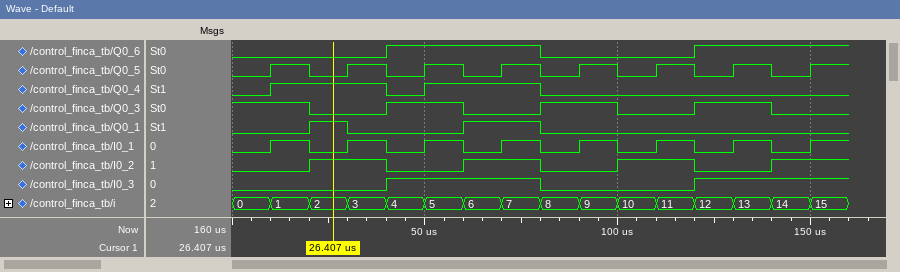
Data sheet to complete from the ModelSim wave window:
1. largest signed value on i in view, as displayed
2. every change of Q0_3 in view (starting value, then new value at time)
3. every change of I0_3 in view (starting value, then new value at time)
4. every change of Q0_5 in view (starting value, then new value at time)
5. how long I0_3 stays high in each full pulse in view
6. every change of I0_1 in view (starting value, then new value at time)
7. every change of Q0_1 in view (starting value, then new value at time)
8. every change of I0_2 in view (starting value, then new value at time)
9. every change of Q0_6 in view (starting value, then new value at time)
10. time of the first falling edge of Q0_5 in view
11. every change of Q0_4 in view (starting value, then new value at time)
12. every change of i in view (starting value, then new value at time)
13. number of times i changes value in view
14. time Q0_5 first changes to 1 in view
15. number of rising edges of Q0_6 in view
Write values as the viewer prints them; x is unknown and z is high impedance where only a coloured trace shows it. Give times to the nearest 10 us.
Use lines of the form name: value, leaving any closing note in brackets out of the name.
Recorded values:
largest signed value on i in view, as displayed: 15
every change of Q0_3 in view: 1, 0 at 20 us, 1 at 40 us, 0 at 60 us, 1 at 80 us, 0 at 100 us, 1 at 120 us, 0 at 140 us
every change of I0_3 in view: 0, 1 at 40 us, 0 at 80 us, 1 at 120 us
every change of Q0_5 in view: 0, 1 at 10 us, 0 at 20 us, 1 at 30 us, 0 at 40 us, 1 at 50 us, 0 at 60 us, 1 at 70 us, 0 at 80 us, 1 at 90 us, 0 at 100 us, 1 at 110 us, 0 at 120 us, 1 at 130 us, 0 at 140 us, 1 at 150 us
how long I0_3 stays high in each full pulse in view: 40 us
every change of I0_1 in view: 0, 1 at 10 us, 0 at 20 us, 1 at 30 us, 0 at 40 us, 1 at 50 us, 0 at 60 us, 1 at 70 us, 0 at 80 us, 1 at 90 us, 0 at 100 us, 1 at 110 us, 0 at 120 us, 1 at 130 us, 0 at 140 us, 1 at 150 us
every change of Q0_1 in view: 0, 1 at 20 us, 0 at 30 us, 1 at 60 us, 0 at 80 us
every change of I0_2 in view: 0, 1 at 20 us, 0 at 40 us, 1 at 60 us, 0 at 80 us, 1 at 100 us, 0 at 120 us, 1 at 140 us
every change of Q0_6 in view: 0, 1 at 40 us, 0 at 80 us, 1 at 120 us
time of the first falling edge of Q0_5 in view: 20 us
every change of Q0_4 in view: 0, 1 at 10 us, 0 at 40 us, 1 at 50 us, 0 at 80 us
every change of i in view: 0, 1 at 10 us, 2 at 20 us, 3 at 30 us, 4 at 40 us, 5 at 50 us, 6 at 60 us, 7 at 70 us, 8 at 80 us, 9 at 90 us, 10 at 100 us, 11 at 110 us, 12 at 120 us, 13 at 130 us, 14 at 140 us, 15 at 150 us
number of times i changes value in view: 15
time Q0_5 first changes to 1 in view: 10 us
number of rising edges of Q0_6 in view: 2
